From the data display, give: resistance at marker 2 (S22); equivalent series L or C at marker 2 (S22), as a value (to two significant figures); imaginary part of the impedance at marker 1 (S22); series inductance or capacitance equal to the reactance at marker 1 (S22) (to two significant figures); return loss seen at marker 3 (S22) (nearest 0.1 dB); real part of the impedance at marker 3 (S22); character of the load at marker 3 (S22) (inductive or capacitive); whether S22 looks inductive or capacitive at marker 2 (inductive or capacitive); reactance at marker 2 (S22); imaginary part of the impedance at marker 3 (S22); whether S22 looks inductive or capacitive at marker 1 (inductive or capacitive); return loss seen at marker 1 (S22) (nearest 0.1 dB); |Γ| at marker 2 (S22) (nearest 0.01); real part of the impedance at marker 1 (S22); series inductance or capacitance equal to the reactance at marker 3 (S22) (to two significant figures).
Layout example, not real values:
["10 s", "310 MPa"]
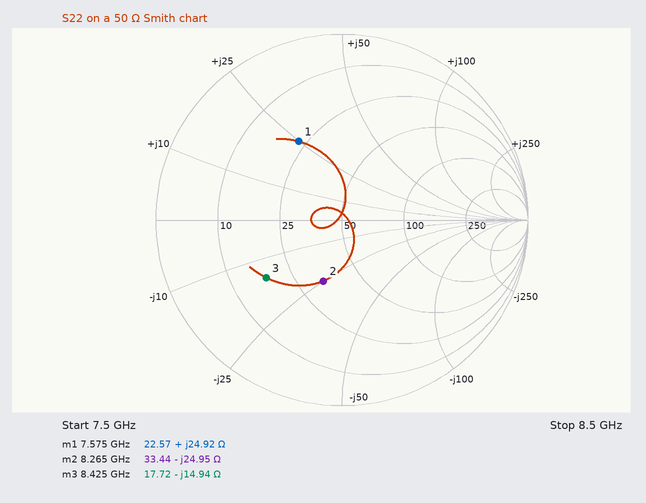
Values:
["33.44 Ω", "770 fF", "+24.92 Ω", "520 pH", "5.8 dB", "17.72 Ω", "capacitive", "capacitive", "-24.95 Ω", "-14.94 Ω", "inductive", "6.3 dB", "0.34", "22.57 Ω", "1.3 pF"]
